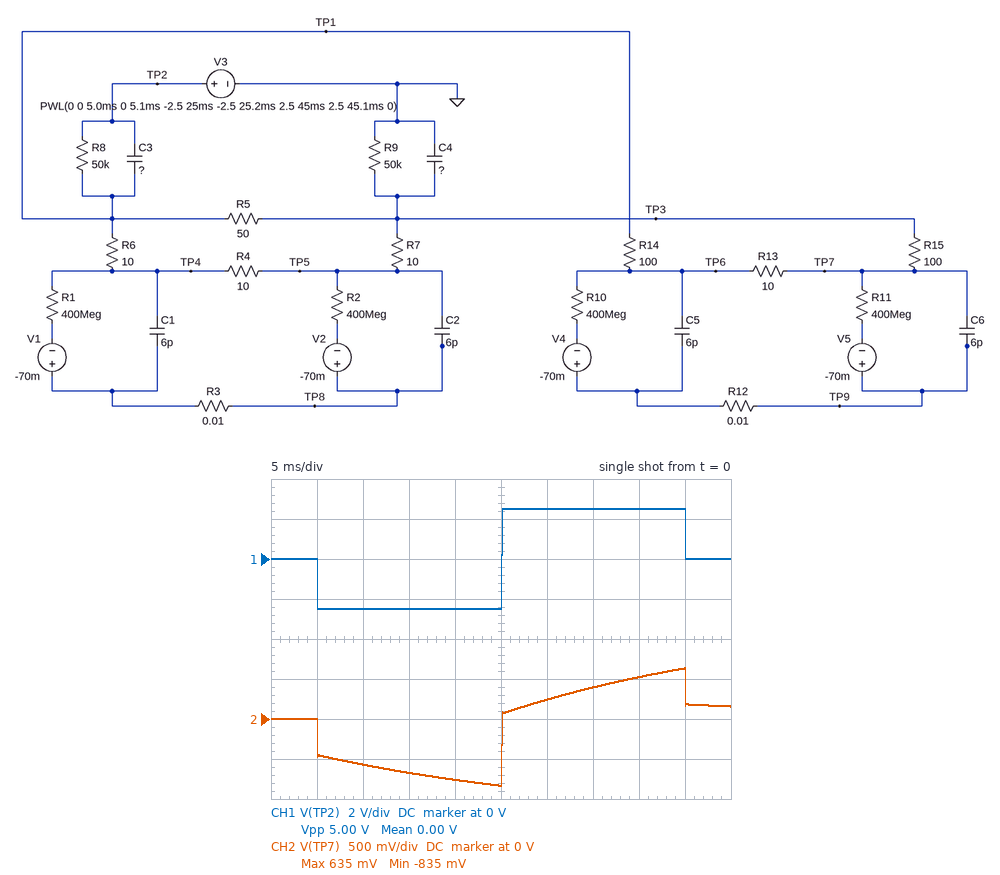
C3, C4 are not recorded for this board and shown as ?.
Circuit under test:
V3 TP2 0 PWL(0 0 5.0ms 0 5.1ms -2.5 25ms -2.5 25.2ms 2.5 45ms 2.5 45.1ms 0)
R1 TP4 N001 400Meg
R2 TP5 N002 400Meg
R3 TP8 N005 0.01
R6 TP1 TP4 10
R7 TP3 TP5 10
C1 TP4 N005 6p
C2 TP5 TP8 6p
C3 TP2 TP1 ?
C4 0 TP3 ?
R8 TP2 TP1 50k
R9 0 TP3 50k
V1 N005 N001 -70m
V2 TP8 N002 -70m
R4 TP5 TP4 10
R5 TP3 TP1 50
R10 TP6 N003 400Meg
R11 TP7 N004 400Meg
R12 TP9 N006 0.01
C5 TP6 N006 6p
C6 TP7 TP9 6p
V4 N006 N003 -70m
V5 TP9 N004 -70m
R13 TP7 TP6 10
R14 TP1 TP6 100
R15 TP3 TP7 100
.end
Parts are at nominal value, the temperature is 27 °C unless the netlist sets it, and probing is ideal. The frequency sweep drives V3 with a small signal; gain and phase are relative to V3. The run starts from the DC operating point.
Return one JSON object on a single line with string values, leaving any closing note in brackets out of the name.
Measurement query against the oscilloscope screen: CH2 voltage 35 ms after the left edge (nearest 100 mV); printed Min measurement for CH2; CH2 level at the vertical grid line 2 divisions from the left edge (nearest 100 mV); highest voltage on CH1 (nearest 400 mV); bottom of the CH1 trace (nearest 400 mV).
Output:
{"CH2 voltage 35 ms after the left edge": "400 mV", "printed Min measurement for CH2": "-835 mV", "CH2 level at the vertical grid line 2 divisions from the left edge": "-600 mV", "highest voltage on CH1": "2.4 V", "bottom of the CH1 trace": "-2.4 V"}
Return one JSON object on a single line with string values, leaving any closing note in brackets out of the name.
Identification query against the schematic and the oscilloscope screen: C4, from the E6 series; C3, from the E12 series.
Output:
{"C4, from the E6 series": "1 µF", "C3, from the E12 series": "220 nF"}
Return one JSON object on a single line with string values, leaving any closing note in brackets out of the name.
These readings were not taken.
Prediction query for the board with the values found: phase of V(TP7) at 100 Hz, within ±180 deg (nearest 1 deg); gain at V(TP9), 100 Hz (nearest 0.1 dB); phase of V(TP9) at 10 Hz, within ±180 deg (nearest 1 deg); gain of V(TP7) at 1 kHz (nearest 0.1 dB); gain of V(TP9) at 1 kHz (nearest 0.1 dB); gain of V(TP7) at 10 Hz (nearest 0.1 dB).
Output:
{"phase of V(TP7) at 100 Hz, within ±180 deg": "-5 deg", "gain at V(TP9), 100 Hz": "-14.8 dB", "phase of V(TP9) at 10 Hz, within ±180 deg": "-28 deg", "gain of V(TP7) at 1 kHz": "-14.9 dB", "gain of V(TP9) at 1 kHz": "-14.9 dB", "gain of V(TP7) at 10 Hz": "-11.0 dB"}
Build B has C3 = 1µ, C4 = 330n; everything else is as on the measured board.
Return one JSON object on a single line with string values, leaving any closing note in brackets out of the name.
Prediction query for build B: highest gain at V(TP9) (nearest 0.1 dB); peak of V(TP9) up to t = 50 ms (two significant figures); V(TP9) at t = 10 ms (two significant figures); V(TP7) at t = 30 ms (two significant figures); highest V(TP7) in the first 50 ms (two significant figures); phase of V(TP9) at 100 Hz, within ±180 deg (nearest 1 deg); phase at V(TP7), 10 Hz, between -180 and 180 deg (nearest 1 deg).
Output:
{"highest gain at V(TP9)": "-2.5 dB", "peak of V(TP9) up to t = 50 ms": "2.1 V", "V(TP9) at t = 10 ms": "-1.9 V", "V(TP7) at t = 30 ms": "2.0 V", "highest V(TP7) in the first 50 ms": "2.2 V", "phase of V(TP9) at 100 Hz, within ±180 deg": "1 deg", "phase at V(TP7), 10 Hz, between -180 and 180 deg": "8 deg"}
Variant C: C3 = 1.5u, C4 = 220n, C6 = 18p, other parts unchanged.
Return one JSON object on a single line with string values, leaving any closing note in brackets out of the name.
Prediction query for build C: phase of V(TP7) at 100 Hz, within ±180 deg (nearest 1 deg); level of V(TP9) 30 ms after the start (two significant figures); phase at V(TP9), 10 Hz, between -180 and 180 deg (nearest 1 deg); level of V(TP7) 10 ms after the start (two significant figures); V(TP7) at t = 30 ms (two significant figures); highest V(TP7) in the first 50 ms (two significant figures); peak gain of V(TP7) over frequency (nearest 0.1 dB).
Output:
{"phase of V(TP7) at 100 Hz, within ±180 deg": "1 deg", "level of V(TP9) 30 ms after the start": "2.3 V", "phase at V(TP9), 10 Hz, between -180 and 180 deg": "8 deg", "level of V(TP7) 10 ms after the start": "-2.1 V", "V(TP7) at t = 30 ms": "2.4 V", "highest V(TP7) in the first 50 ms": "2.5 V", "peak gain of V(TP7) over frequency": "-1.2 dB"}
